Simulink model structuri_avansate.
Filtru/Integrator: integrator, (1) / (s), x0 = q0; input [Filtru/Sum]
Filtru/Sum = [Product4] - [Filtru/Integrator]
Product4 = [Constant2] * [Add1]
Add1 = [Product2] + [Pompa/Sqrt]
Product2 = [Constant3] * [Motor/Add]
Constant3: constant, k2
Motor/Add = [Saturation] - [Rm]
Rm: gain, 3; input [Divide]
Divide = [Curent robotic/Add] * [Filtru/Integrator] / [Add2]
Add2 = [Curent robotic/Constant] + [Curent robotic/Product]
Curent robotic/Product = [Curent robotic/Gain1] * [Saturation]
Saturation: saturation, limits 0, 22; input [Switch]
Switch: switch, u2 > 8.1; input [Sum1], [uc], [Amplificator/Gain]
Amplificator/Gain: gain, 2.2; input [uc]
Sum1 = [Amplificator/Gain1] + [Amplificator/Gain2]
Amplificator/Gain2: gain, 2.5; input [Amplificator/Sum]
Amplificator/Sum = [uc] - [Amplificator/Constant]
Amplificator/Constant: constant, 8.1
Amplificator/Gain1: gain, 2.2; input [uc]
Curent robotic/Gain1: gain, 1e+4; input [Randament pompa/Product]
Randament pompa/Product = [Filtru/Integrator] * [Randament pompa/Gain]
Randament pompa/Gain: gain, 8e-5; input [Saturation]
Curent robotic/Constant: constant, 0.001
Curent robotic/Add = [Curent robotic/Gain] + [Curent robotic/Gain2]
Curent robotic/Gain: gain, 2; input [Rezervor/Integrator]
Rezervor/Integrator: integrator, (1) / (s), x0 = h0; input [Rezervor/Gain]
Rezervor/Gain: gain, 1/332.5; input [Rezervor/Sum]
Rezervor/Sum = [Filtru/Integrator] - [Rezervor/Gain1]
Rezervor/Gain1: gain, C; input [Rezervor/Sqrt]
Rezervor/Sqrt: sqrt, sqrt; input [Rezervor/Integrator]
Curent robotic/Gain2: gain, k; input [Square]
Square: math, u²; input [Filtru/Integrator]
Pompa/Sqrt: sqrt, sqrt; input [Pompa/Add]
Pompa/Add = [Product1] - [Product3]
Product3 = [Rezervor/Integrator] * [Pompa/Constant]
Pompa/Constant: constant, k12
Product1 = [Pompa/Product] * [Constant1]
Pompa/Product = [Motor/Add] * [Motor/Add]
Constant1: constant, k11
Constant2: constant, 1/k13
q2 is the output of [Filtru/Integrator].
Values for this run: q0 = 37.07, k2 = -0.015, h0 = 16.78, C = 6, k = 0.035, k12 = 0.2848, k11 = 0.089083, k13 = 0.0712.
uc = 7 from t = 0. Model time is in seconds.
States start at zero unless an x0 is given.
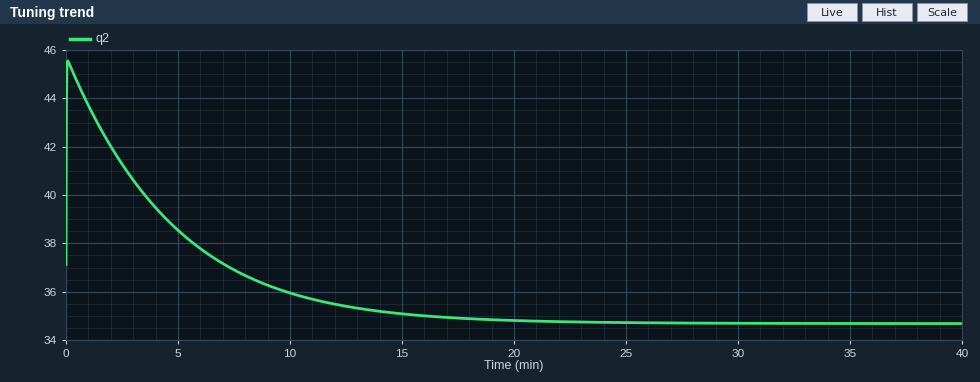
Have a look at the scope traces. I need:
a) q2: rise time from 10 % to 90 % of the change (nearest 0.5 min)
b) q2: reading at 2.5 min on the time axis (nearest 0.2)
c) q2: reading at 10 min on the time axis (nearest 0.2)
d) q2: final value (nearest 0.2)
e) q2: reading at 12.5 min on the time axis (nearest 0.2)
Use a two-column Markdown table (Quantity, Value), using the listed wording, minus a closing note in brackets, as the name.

| Quantity | Value |
|---|---|
| q2: rise time from 10 % to 90 % of the change | 9.5 min |
| q2: reading at 2.5 min on the time axis | 41.2 |
| q2: reading at 10 min on the time axis | 36.0 |
| q2: final value | 34.6 |
| q2: reading at 12.5 min on the time axis | 35.4 |
